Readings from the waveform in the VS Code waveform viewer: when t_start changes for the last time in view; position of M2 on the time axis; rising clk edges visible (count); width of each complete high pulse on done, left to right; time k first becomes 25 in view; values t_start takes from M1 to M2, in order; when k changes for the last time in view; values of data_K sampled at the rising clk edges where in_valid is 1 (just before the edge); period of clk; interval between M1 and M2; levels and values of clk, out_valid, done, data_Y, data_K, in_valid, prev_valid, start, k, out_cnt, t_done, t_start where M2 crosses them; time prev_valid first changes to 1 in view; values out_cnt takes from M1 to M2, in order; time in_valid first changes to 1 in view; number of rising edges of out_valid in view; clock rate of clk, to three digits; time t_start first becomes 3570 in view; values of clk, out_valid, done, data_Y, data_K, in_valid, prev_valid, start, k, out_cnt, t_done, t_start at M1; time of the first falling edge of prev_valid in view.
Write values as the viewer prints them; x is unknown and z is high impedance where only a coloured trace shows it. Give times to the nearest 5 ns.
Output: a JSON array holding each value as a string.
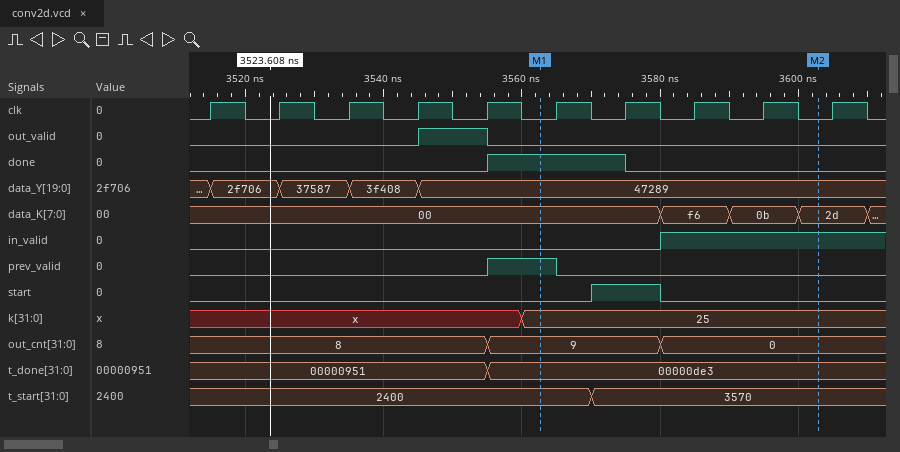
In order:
["3570 ns", "3605 ns", "10", "20 ns", "3560 ns", "2400, 3570", "3560 ns", "f6, 0b, 2d", "10 ns", "40 ns", "clk=0, out_valid=0, done=0, data_Y=47289, data_K=2d, in_valid=1, prev_valid=0, start=0, k=25, out_cnt=0, t_done=00000de3, t_start=3570", "3555 ns", "9, 0", "3580 ns", "1", "100 MHz", "3570 ns", "clk=0, out_valid=0, done=1, data_Y=47289, data_K=00, in_valid=0, prev_valid=1, start=0, k=25, out_cnt=9, t_done=00000de3, t_start=2400", "3565 ns"]
